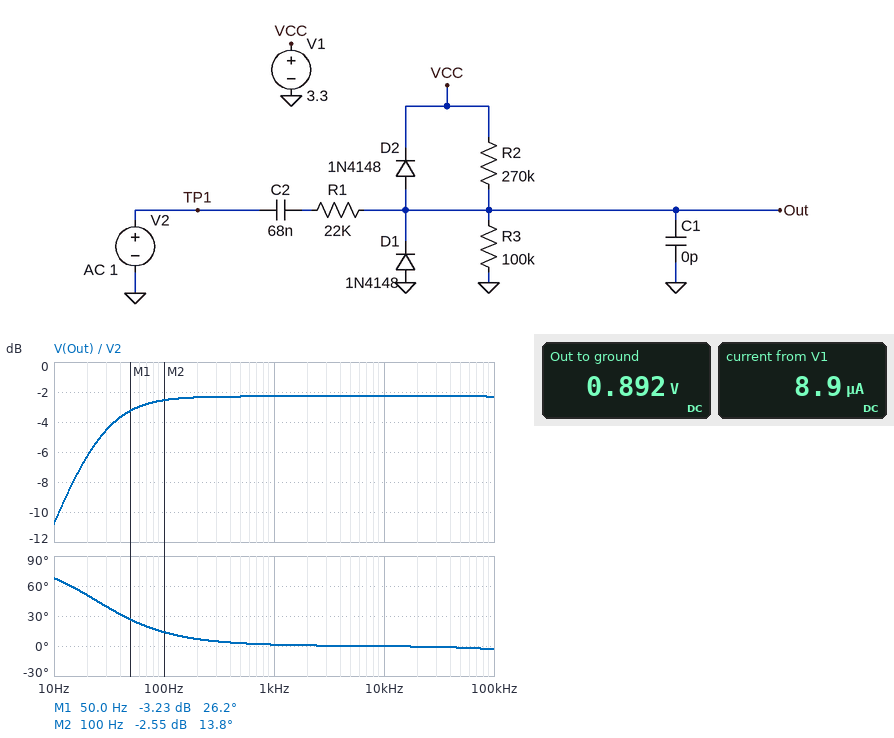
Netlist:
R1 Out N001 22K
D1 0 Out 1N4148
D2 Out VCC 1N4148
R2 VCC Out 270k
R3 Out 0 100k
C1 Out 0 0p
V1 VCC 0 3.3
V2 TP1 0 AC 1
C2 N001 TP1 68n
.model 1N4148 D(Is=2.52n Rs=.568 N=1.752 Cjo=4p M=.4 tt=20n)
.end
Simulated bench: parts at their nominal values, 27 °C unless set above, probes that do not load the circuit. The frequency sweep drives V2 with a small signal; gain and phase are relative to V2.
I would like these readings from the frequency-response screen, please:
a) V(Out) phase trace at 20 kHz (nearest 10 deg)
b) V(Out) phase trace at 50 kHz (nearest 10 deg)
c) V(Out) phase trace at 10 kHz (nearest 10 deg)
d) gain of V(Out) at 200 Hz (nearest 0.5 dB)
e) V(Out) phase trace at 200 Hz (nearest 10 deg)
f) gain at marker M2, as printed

0 deg
0 deg
0 deg
-2.5 dB
10 deg
-2.55 dB
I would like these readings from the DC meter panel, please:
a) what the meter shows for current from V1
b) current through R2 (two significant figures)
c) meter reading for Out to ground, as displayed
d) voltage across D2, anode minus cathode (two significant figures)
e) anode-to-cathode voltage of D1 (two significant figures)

8.9 µA
8.9 µA
0.892 V
-2.4 V
-890 mV
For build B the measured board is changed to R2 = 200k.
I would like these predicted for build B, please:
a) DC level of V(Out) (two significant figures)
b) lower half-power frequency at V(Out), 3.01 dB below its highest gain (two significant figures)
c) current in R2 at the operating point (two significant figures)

1.1 V
26 Hz
11 µA
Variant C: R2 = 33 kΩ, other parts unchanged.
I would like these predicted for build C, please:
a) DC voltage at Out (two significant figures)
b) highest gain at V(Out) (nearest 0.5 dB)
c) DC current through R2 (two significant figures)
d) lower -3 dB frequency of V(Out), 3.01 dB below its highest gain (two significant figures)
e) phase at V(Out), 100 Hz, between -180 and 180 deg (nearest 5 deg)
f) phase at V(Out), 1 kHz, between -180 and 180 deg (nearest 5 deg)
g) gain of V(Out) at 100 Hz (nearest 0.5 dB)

2.5 V
-5.5 dB
25 µA
50 Hz
25 deg
5 deg
-6.5 dB
